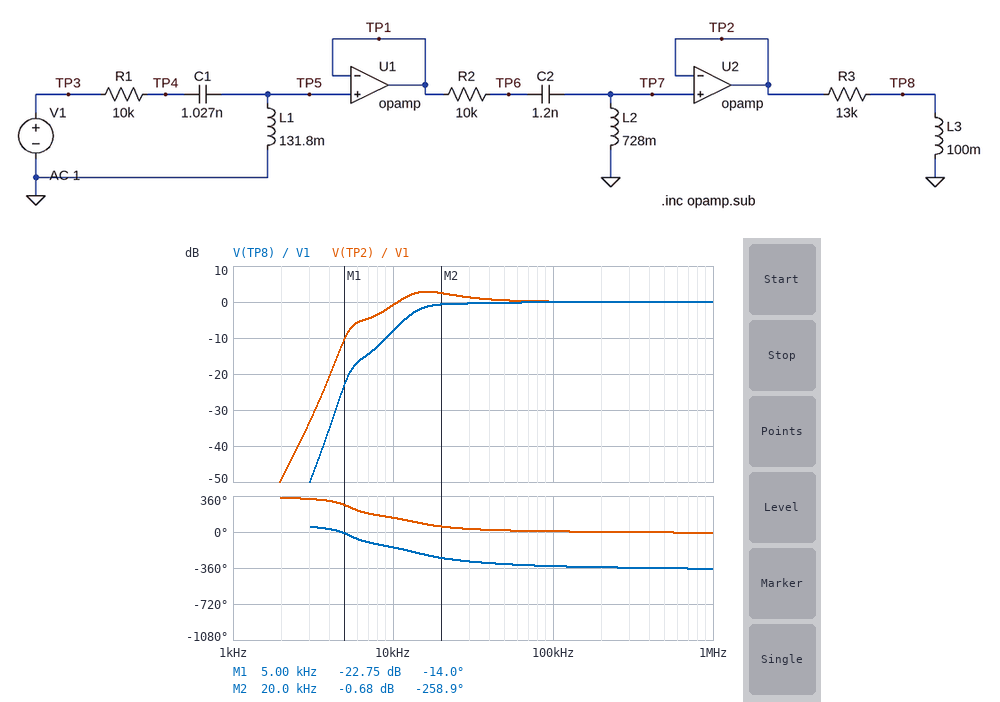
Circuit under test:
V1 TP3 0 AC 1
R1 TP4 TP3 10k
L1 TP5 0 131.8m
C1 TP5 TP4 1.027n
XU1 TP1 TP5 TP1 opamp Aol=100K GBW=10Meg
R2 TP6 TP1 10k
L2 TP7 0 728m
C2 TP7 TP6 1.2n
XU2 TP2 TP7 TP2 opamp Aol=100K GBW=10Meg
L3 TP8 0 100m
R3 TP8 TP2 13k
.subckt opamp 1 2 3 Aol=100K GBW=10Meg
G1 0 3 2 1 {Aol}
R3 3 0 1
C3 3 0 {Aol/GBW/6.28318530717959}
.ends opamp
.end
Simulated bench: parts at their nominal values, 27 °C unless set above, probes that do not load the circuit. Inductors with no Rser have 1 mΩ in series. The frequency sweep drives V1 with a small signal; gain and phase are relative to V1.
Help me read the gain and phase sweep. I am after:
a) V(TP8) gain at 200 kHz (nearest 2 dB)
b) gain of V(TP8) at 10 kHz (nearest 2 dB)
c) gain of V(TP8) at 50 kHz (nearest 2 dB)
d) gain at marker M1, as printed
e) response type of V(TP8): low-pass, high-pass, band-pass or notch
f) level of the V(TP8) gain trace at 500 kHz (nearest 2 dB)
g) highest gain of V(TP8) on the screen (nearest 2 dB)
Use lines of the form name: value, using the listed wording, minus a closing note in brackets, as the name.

V(TP8) gain at 200 kHz: 0 dB
gain of V(TP8) at 10 kHz: -8 dB
gain of V(TP8) at 50 kHz: 0 dB
gain at marker M1, as printed: -22.75 dB
response type of V(TP8): low-pass, high-pass, band-pass or notch: high-pass
level of the V(TP8) gain trace at 500 kHz: 0 dB
highest gain of V(TP8) on the screen: 0 dB
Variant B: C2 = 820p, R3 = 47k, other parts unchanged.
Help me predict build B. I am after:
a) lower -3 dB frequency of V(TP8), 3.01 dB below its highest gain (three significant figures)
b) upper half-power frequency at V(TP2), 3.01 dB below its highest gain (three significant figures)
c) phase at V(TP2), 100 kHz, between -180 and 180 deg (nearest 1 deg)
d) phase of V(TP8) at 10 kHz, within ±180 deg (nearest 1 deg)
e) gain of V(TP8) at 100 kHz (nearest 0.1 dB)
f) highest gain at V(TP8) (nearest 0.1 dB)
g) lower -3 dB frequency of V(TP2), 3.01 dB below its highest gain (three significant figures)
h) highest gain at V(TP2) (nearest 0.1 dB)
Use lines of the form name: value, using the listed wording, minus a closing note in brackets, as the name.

lower -3 dB frequency of V(TP8), 3.01 dB below its highest gain: 68.9 kHz
upper half-power frequency at V(TP2), 3.01 dB below its highest gain: 58.8 kHz
phase at V(TP2), 100 kHz, between -180 and 180 deg: 7 deg
phase of V(TP8) at 10 kHz, within ±180 deg: -131 deg
gain of V(TP8) at 100 kHz: -1.8 dB
highest gain at V(TP8): -0.1 dB
lower -3 dB frequency of V(TP2), 3.01 dB below its highest gain: 9.55 kHz
highest gain at V(TP2): 3.4 dB
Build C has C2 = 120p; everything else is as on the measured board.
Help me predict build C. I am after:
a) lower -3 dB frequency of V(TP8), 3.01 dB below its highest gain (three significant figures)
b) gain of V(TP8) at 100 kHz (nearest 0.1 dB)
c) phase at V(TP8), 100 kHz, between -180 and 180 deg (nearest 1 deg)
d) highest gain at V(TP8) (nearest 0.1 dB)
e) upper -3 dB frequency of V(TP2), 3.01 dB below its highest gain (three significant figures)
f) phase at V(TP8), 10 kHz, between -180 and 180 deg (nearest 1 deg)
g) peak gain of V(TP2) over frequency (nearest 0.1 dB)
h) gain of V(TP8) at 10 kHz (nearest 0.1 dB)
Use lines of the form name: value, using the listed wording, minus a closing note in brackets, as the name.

lower -3 dB frequency of V(TP8), 3.01 dB below its highest gain: 16.2 kHz
gain of V(TP8) at 100 kHz: 0.2 dB
phase at V(TP8), 100 kHz, between -180 and 180 deg: 19 deg
highest gain at V(TP8): 16.0 dB
upper -3 dB frequency of V(TP2), 3.01 dB below its highest gain: 18.3 kHz
phase at V(TP8), 10 kHz, between -180 and 180 deg: 3 deg
peak gain of V(TP2) over frequency: 19.9 dB
gain of V(TP8) at 10 kHz: -16.3 dB
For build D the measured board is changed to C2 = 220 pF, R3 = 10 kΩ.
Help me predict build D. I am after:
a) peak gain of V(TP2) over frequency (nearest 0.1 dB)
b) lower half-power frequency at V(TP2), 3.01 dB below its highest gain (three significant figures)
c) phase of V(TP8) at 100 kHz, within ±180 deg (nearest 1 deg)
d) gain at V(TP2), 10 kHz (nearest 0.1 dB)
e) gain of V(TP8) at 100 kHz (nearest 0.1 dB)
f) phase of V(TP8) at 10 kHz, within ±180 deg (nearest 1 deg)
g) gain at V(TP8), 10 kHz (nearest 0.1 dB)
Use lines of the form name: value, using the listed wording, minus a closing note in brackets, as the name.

peak gain of V(TP2) over frequency: 15.6 dB
lower half-power frequency at V(TP2), 3.01 dB below its highest gain: 11.9 kHz
phase of V(TP8) at 100 kHz, within ±180 deg: 16 deg
gain at V(TP2), 10 kHz: 0.7 dB
gain of V(TP8) at 100 kHz: 0.1 dB
phase of V(TP8) at 10 kHz, within ±180 deg: -17 deg
gain at V(TP8), 10 kHz: -4.8 dB
